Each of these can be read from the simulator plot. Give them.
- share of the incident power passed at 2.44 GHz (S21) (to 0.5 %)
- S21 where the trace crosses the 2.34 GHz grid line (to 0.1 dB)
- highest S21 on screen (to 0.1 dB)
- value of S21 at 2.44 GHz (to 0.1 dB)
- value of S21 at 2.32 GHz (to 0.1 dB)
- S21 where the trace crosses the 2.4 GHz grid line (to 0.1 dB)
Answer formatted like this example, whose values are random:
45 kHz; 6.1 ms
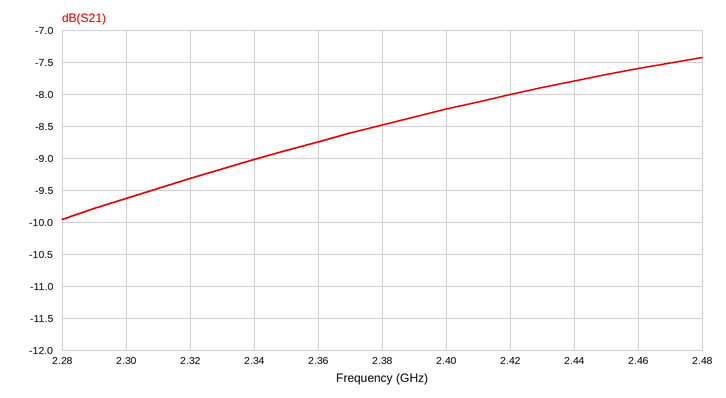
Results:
16.5 %; -9.0 dB; -7.4 dB; -7.8 dB; -9.3 dB; -8.2 dB
